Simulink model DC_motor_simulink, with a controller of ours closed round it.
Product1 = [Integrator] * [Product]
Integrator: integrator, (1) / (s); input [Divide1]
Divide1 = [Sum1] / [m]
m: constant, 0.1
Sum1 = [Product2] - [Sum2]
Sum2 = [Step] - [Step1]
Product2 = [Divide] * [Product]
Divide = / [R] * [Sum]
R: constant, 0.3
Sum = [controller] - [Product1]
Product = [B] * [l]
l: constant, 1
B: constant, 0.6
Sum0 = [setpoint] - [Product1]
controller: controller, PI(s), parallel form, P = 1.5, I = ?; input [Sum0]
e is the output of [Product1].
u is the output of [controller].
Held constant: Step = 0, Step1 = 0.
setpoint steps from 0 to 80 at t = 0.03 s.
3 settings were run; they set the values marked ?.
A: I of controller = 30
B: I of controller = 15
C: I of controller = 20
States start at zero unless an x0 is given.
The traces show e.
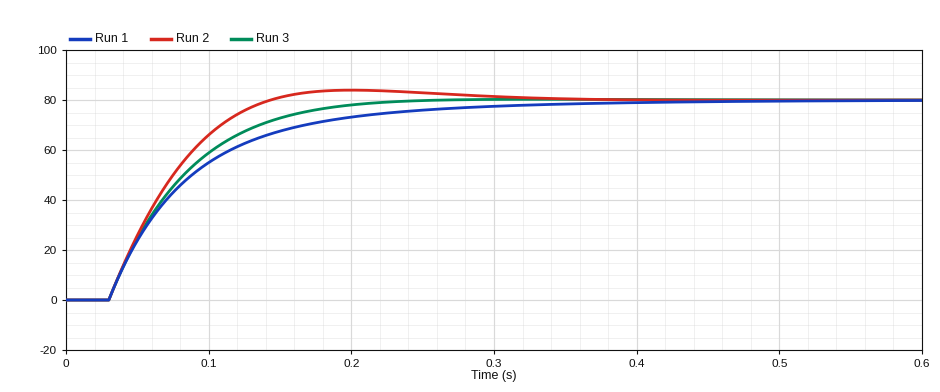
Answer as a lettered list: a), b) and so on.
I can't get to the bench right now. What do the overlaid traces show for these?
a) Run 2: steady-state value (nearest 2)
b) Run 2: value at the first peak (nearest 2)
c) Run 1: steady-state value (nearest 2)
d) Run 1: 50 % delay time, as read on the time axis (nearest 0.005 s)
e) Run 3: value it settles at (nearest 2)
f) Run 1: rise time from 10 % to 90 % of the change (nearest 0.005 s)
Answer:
a) 80
b) 84
c) 80
d) 0.070 s
e) 80
f) 0.150 s
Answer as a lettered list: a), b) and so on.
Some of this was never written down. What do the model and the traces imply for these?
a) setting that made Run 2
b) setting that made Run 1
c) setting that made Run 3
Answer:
a) A
b) B
c) C
